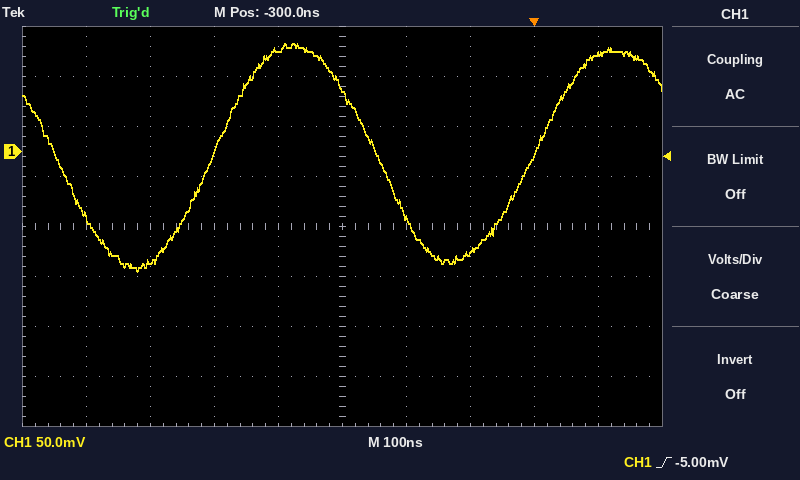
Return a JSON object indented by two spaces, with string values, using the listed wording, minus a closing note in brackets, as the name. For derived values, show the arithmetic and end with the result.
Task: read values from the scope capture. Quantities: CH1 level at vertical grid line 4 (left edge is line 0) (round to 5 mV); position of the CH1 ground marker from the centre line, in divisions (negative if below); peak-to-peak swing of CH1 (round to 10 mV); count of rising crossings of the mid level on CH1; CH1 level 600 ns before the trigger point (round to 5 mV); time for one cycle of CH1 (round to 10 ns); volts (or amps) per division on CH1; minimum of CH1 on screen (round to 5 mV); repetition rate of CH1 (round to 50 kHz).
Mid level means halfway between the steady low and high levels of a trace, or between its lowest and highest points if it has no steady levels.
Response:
{
  "CH1 level at vertical grid line 4 (left edge is line 0)": "100 mV",
  "position of the CH1 ground marker from the centre line, in divisions": "+1.5 div",
  "peak-to-peak swing of CH1": "230 mV",
  "count of rising crossings of the mid level on CH1": "2",
  "CH1 level 600 ns before the trigger point": "-110 mV",
  "time for one cycle of CH1": "500 ns",
  "volts (or amps) per division on CH1": "50 mV",
  "minimum of CH1 on screen": "-120 mV",
  "repetition rate of CH1": "1 / 500 ns ≈ 2.00 MHz"
}
